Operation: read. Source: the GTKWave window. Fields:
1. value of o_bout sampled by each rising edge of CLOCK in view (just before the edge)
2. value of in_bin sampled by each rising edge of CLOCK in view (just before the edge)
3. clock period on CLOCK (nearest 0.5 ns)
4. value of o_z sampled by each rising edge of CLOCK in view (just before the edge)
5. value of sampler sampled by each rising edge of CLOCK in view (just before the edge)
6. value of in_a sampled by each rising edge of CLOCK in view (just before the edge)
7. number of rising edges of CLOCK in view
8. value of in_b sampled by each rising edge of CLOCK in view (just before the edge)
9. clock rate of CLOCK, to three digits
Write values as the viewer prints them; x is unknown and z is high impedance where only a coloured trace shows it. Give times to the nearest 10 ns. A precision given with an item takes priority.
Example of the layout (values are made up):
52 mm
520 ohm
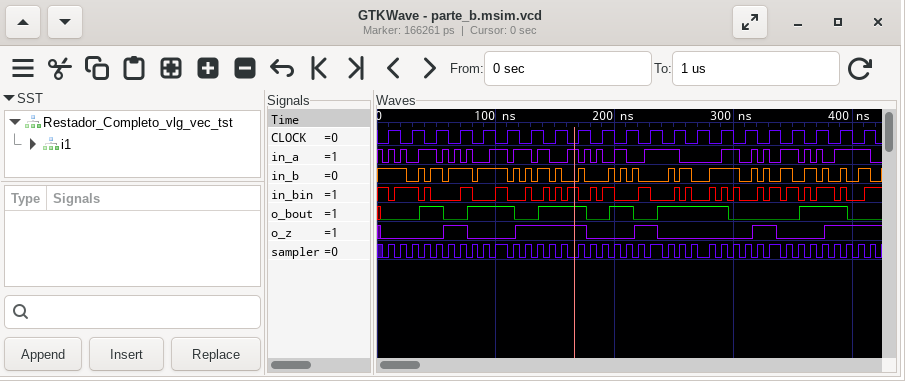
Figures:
0 0 1 0 1 1 0 1 1 0 1 0 1 1 1 0 0 0 1 1 0
1 1 0 0 0 1 1 0 1 0 0 1 0 0 0 0 0 1 0 0 0
20 ns
0 0 0 1 0 0 1 1 1 0 0 1 0 0 0 0 1 0 0 1 1
0 0 0 0 0 1 1 1 0 0 0 0 1 1 0 0 0 1 1 1 1
0 0 1 1 0 1 1 0 1 1 1 1 1 0 0 0 1 1 0 1 1
21
1 0 1 1 1 1 1 0 0 0 1 0 1 0 1 0 1 1 1 0 1
50.0 MHz
